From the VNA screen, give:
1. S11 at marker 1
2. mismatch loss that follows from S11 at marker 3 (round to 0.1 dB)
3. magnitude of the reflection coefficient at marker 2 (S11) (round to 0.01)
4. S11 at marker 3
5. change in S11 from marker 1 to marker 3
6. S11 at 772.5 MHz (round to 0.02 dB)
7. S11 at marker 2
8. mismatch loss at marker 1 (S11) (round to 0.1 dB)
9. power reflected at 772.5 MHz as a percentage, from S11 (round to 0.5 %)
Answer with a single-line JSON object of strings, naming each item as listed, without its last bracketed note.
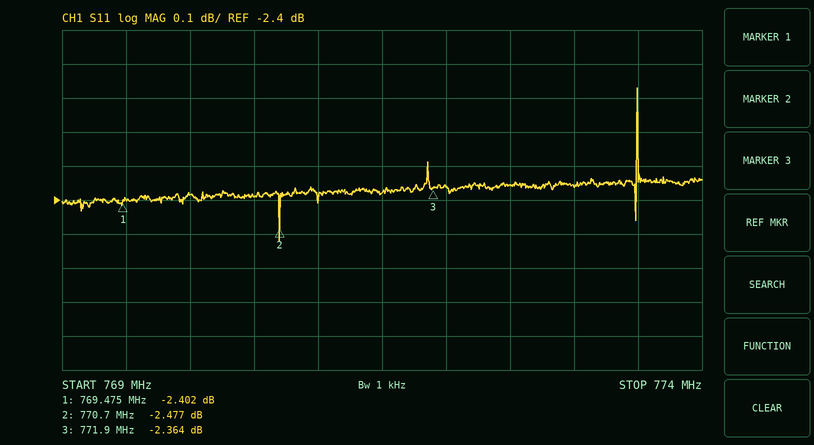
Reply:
{"S11 at marker 1": "-2.402 dB", "mismatch loss that follows from S11 at marker 3": "3.8 dB", "magnitude of the reflection coefficient at marker 2 (S11)": "0.75", "S11 at marker 3": "-2.364 dB", "change in S11 from marker 1 to marker 3": "0.038 dB", "S11 at 772.5 MHz": "-2.36 dB", "S11 at marker 2": "-2.477 dB", "mismatch loss at marker 1 (S11)": "3.7 dB", "power reflected at 772.5 MHz as a percentage, from S11": "58.0 %"}
